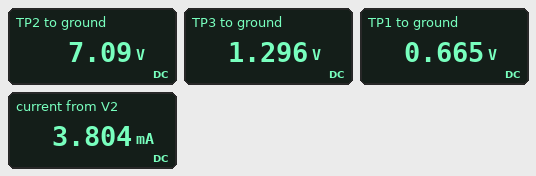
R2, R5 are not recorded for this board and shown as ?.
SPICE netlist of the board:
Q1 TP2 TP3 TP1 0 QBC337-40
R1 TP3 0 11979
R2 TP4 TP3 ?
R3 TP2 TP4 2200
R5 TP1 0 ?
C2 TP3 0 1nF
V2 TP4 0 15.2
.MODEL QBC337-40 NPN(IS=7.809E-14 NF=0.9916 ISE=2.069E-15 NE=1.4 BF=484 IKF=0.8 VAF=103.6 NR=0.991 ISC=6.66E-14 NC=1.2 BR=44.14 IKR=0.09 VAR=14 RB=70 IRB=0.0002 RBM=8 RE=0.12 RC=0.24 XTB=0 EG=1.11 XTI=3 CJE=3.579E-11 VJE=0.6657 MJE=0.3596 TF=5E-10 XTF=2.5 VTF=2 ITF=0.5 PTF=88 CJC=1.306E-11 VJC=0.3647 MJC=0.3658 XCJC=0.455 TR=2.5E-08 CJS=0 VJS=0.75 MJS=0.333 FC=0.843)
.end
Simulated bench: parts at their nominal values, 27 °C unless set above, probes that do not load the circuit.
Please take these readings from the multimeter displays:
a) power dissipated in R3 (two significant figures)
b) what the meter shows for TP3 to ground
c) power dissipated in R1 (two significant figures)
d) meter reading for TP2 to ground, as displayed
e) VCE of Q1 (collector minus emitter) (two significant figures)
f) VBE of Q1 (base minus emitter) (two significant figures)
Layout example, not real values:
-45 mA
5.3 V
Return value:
30 mW
1.296 V
140 µW
7.09 V
6.4 V
630 mV
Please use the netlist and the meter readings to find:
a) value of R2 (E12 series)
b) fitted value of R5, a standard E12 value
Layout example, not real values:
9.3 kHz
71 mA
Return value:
120 kΩ
180 Ω
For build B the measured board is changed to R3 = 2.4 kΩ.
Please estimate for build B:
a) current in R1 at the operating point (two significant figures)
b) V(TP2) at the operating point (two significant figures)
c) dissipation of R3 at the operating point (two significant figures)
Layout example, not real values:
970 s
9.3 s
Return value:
110 µA
6.4 V
33 mW
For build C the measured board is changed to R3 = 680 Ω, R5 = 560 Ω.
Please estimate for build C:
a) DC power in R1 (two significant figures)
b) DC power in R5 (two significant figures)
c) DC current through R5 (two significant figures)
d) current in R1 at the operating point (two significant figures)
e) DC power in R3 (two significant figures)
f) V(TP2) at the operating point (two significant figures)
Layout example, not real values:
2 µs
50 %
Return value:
150 µW
1.0 mW
1.3 mA
110 µA
1.2 mW
14 V
